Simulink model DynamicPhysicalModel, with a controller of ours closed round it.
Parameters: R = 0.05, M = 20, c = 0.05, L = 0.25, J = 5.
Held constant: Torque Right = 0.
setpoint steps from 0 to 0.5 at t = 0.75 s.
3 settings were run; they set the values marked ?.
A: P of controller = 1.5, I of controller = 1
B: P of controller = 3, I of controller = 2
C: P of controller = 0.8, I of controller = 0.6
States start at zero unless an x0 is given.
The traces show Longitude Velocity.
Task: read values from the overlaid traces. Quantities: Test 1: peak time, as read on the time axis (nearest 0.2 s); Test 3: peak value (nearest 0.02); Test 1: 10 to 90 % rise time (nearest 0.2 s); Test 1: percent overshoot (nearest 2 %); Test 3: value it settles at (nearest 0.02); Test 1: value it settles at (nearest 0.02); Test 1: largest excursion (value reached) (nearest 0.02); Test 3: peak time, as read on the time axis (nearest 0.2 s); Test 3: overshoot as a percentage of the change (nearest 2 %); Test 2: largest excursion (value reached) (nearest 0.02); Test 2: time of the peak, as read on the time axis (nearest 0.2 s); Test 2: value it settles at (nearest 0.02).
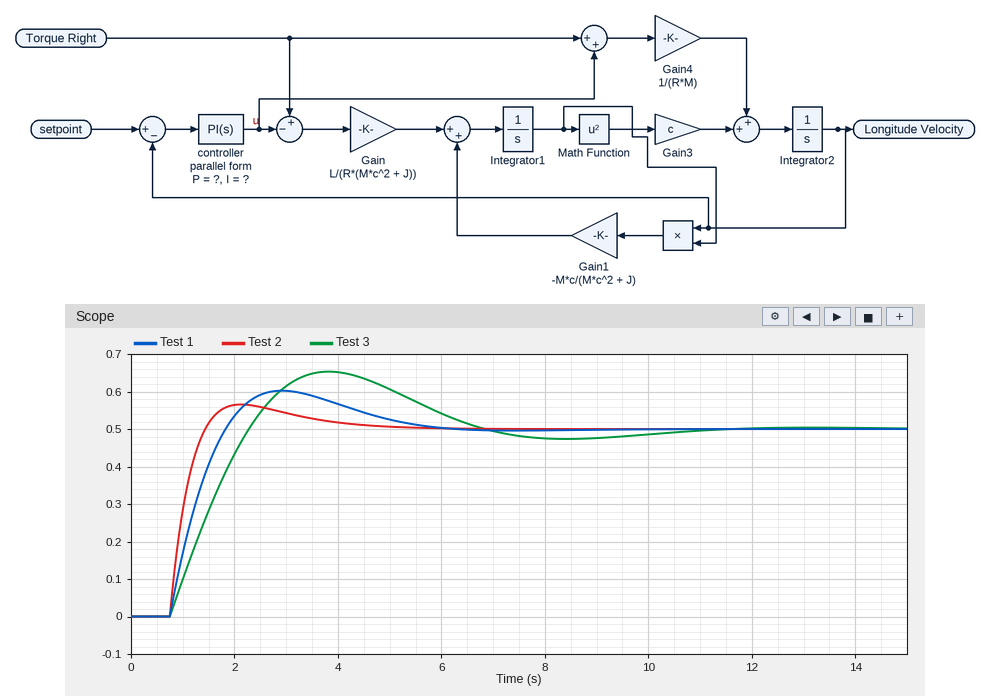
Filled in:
3.0 s
0.66
0.8 s
20 %
0.50
0.50
0.60
3.8 s
30 %
0.56
2.2 s
0.50
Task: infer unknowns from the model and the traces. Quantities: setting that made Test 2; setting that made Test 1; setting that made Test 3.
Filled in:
B
A
C
